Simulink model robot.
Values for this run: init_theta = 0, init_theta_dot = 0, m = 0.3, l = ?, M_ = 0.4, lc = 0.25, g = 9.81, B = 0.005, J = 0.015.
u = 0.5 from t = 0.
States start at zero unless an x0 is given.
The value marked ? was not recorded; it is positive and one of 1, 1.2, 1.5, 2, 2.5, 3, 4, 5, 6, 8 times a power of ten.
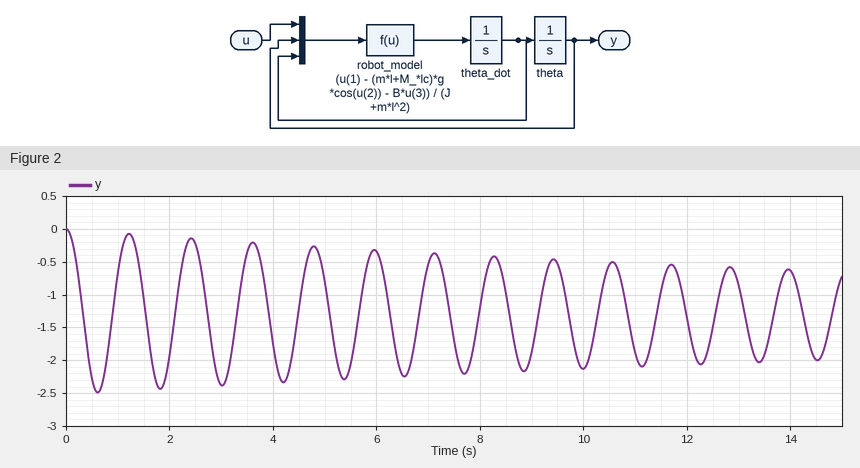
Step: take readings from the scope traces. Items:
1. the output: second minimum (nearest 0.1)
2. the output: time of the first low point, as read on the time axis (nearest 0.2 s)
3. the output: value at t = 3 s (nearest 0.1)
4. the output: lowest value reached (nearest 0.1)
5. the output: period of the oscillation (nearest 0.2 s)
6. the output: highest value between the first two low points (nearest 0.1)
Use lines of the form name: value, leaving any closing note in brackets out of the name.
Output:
the output: second minimum: -2.4
the output: time of the first low point, as read on the time axis: 0.6 s
the output: value at t = 3 s: -2.4
the output: lowest value reached: -2.5
the output: period of the oscillation: 1.2 s
the output: highest value between the first two low points: -0.1
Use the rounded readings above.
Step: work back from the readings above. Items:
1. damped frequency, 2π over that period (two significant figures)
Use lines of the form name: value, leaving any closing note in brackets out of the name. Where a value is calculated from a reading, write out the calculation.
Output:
damped frequency, 2π over that period: 2π / 1.2 = 5.2 rad/s
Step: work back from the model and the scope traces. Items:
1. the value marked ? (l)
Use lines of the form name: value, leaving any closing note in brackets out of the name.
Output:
the value marked ?: 0.4
